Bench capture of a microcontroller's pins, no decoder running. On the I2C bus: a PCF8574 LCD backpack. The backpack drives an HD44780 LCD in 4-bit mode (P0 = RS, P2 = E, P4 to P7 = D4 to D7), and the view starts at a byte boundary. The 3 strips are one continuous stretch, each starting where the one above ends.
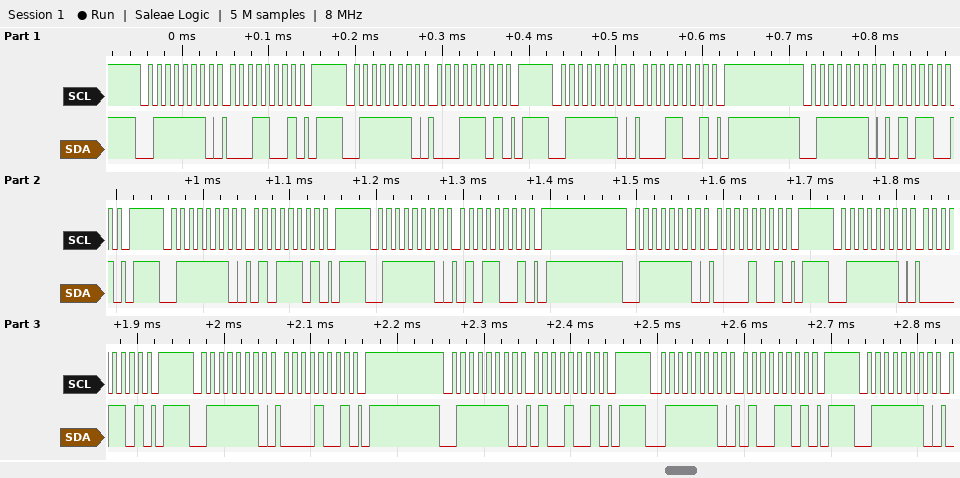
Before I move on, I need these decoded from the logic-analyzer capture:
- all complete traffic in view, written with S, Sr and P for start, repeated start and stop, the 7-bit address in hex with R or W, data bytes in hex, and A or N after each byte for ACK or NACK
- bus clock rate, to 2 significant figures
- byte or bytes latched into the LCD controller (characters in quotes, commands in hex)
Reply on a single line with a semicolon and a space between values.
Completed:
S 3FW A 19 A P S 3FW A 1D A P S 3FW A 19 A P S 3FW A 59 A P S 3FW A 5D A P S 3FW A 59 A P S 3FW A 09 A P S 3FW A 0D A P S 3FW A 09 A P S 3FW A 49 A P S 3FW A 4D A P S 3FW A; 100 kHz; data 0x15
